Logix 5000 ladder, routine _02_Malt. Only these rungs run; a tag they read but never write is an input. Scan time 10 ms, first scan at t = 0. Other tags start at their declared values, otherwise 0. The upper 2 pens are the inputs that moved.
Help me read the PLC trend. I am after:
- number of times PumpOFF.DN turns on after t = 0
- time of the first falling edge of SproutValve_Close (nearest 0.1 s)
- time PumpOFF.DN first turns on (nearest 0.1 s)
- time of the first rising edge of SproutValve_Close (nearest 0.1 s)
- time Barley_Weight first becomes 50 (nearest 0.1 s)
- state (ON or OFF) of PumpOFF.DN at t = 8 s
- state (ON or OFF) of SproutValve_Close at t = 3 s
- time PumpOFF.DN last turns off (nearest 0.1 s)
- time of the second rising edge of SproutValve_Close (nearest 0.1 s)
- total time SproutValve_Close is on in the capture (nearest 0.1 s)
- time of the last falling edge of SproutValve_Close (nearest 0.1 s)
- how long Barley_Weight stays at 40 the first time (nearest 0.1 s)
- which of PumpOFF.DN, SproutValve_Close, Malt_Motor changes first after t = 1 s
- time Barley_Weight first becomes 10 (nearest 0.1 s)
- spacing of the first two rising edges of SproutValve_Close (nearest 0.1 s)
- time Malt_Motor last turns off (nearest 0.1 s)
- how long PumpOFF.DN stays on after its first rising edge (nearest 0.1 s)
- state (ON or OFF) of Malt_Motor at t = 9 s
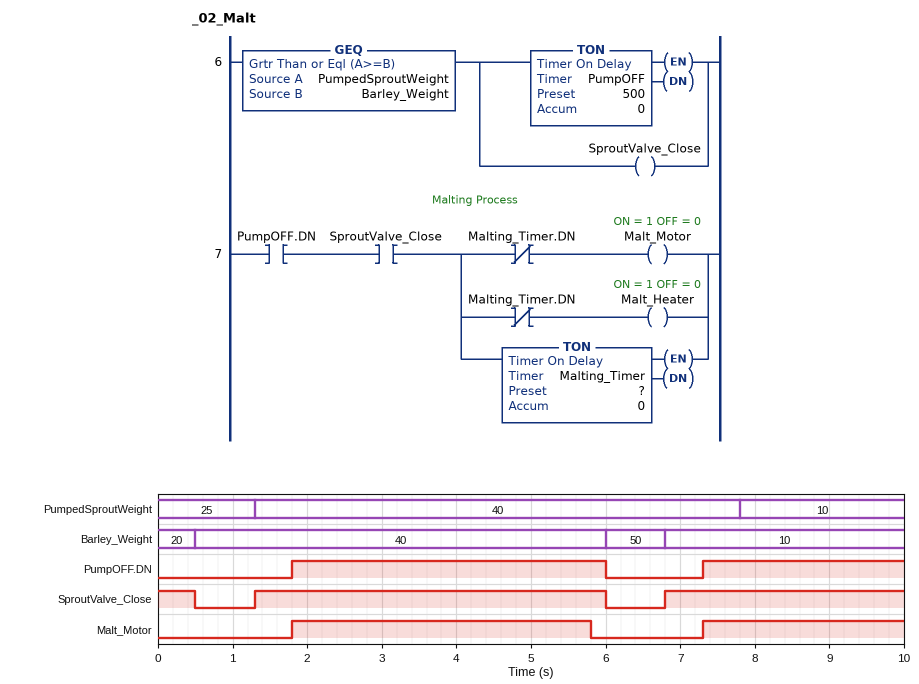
2
0.5 s
1.8 s
1.3 s
6.0 s
ON
ON
6.0 s
6.8 s
8.4 s
6.0 s
5.5 s
SproutValve_Close
6.8 s
5.5 s
5.8 s
4.2 s
ON
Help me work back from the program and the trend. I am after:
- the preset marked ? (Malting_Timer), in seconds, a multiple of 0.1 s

4.0 s
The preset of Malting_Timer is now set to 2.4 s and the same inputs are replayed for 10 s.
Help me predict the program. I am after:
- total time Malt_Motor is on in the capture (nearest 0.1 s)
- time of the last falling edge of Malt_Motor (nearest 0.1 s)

4.8 s
9.7 s
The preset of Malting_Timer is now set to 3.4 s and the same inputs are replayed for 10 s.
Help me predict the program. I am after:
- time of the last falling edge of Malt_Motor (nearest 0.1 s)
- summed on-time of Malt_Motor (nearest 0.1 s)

5.2 s
6.1 s
